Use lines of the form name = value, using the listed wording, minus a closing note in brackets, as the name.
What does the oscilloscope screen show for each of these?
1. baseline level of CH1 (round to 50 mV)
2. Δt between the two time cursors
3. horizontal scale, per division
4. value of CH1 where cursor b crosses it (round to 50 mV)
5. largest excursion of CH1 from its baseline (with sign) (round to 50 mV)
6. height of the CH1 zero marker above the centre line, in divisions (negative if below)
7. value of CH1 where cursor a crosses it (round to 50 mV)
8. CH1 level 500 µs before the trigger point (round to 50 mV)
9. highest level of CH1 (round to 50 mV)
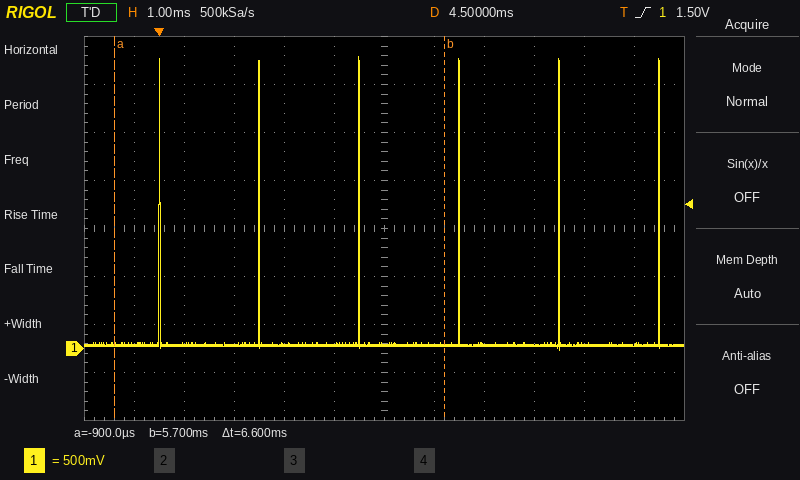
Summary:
baseline level of CH1 = 50 mV
Δt between the two time cursors = 6.6 ms
horizontal scale, per division = 1 ms
value of CH1 where cursor b crosses it = 50 mV
largest excursion of CH1 from its baseline (with sign) = +3.00 V
height of the CH1 zero marker above the centre line, in divisions = -2.5 div
value of CH1 where cursor a crosses it = 50 mV
CH1 level 500 µs before the trigger point = 50 mV
highest level of CH1 = 3.05 V
